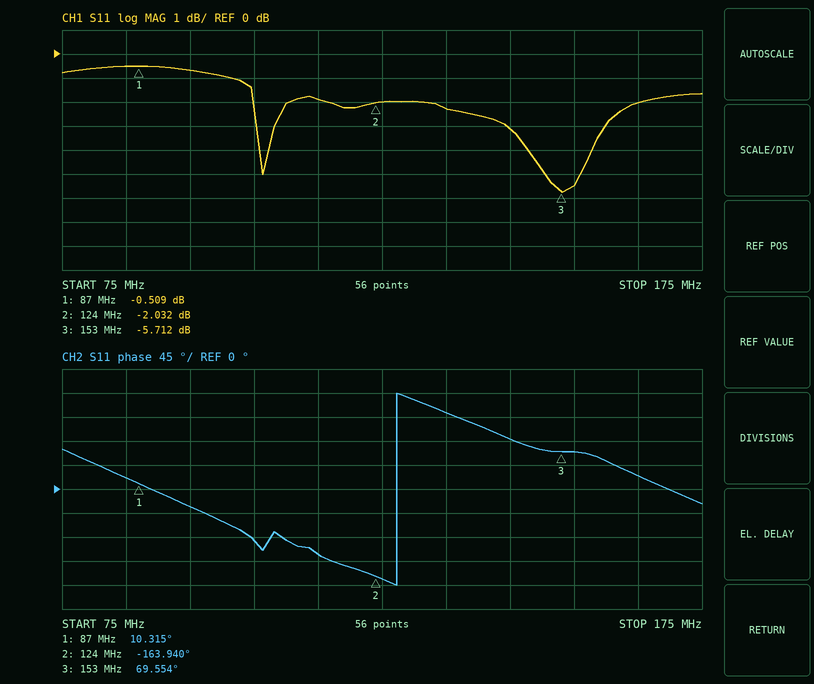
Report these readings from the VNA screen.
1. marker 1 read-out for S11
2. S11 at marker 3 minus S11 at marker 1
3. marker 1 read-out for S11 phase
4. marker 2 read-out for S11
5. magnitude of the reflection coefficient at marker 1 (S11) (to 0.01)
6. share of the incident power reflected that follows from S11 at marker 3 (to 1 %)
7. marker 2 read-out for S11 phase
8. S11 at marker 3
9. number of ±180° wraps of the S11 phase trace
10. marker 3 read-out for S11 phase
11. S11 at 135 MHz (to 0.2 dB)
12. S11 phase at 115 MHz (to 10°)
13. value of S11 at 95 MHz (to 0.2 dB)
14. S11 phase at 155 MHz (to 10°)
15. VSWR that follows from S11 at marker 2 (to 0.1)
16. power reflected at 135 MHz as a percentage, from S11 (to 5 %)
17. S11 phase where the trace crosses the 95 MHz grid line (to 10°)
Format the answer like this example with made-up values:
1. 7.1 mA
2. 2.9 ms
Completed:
1. -0.509 dB
2. -5.203 dB
3. 10.315°
4. -2.032 dB
5. 0.94
6. 27 %
7. -163.940°
8. -5.712 dB
9. 1
10. 69.554°
11. -2.2 dB
12. -120°
13. -0.6 dB
14. 70°
15. 8.6
16. 60 %
17. -30°
